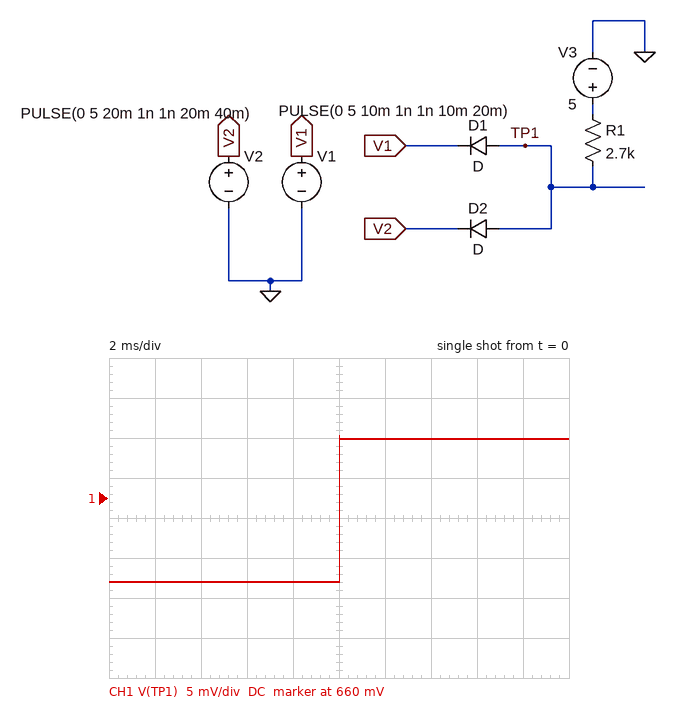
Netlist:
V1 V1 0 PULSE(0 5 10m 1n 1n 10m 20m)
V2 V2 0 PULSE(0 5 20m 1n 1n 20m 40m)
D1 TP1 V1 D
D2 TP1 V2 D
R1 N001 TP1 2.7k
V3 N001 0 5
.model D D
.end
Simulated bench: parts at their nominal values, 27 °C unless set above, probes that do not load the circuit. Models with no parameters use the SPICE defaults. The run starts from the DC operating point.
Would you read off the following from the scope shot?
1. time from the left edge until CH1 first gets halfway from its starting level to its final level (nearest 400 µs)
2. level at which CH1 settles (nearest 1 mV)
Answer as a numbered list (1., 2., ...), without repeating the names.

1. 10.0 ms
2. 667 mV
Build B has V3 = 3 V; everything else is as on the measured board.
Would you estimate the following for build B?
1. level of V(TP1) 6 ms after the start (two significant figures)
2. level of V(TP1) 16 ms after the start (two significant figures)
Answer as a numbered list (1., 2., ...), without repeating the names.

1. 630 mV
2. 650 mV
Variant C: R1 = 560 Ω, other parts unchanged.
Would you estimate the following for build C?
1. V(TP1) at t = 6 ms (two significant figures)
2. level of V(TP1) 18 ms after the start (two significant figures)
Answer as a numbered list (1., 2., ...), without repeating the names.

1. 690 mV
2. 710 mV
